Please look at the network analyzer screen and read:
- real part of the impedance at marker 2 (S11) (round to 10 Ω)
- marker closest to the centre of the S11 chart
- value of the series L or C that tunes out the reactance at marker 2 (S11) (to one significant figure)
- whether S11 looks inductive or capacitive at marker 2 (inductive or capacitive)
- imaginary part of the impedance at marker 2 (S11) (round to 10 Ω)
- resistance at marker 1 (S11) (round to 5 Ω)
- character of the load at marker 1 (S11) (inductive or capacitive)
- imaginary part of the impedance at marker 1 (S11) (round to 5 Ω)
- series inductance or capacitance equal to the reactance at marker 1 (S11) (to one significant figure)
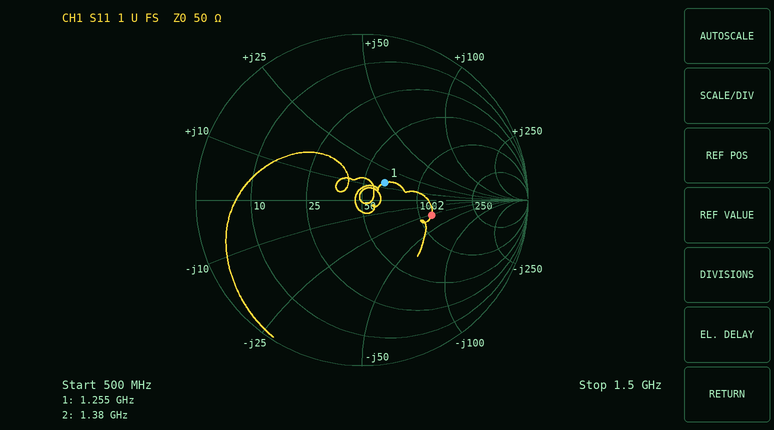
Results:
120 Ω
marker 1
3 nH
capacitive
-30 Ω
65 Ω
inductive
+15 Ω
2 nH
